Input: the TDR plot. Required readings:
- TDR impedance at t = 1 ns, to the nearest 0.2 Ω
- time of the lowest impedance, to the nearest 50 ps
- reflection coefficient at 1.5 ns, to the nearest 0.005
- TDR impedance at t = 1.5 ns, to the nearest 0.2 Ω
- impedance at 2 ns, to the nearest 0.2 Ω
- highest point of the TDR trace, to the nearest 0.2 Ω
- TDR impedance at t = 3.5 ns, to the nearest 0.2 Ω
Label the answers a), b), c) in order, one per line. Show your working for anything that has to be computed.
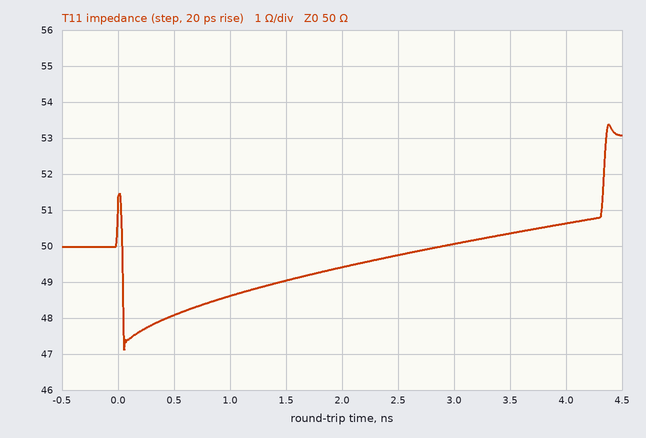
a) 48.6 Ω
b) 50 ps
c) (49 − 50)/(49 + 50) ≈ -0.010
d) 49.0 Ω
e) 49.4 Ω
f) 53.4 Ω
g) 50.4 Ω
